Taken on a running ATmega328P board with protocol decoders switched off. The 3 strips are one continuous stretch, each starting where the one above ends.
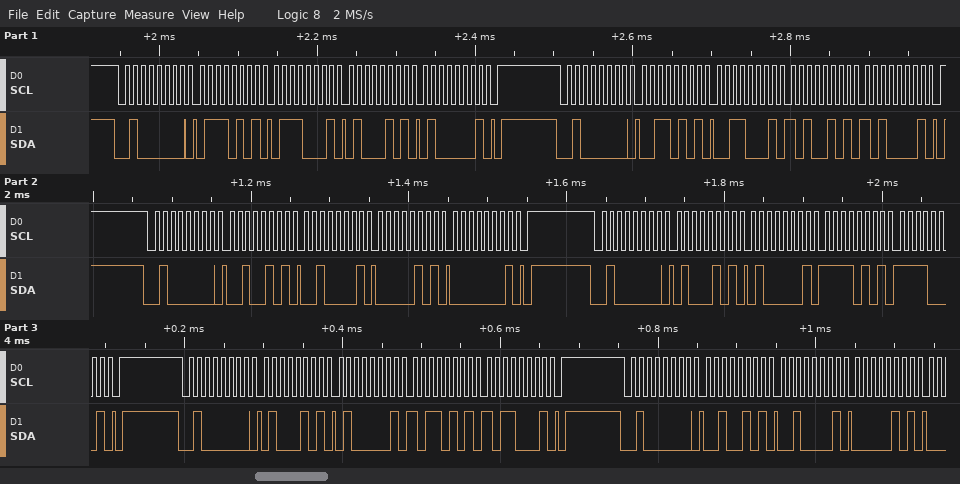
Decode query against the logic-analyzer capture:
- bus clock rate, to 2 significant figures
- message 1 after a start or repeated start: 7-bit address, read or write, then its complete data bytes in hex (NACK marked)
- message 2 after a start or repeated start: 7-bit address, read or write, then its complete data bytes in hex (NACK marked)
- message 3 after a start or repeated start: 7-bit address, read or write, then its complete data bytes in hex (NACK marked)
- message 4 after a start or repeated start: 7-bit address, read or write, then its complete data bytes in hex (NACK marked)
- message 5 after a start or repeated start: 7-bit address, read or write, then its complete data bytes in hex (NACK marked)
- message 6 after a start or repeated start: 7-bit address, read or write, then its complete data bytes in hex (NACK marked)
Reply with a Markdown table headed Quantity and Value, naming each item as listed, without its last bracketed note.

| Quantity | Value |
|---|---|
| bus clock rate, to 2 significant figures | 100 kHz |
| message 1 after a start or repeated start: 7-bit address, read or write, then its complete data bytes in hex | 0x20 write: 75 71 45 41 |
| message 2 after a start or repeated start: 7-bit address, read or write, then its complete data bytes in hex | 0x20 write: 35 31 A5 A1 |
| message 3 after a start or repeated start: 7-bit address, read or write, then its complete data bytes in hex | 0x20 write: 25 21 05 01 |
| message 4 after a start or repeated start: 7-bit address, read or write, then its complete data bytes in hex | 0x20 write: 45 41 F5 F1 |
| message 5 after a start or repeated start: 7-bit address, read or write, then its complete data bytes in hex | 0x20 write: 45 41 B5 B1 |
| message 6 after a start or repeated start: 7-bit address, read or write, then its complete data bytes in hex | 0x20 write: 25 21 05 |
